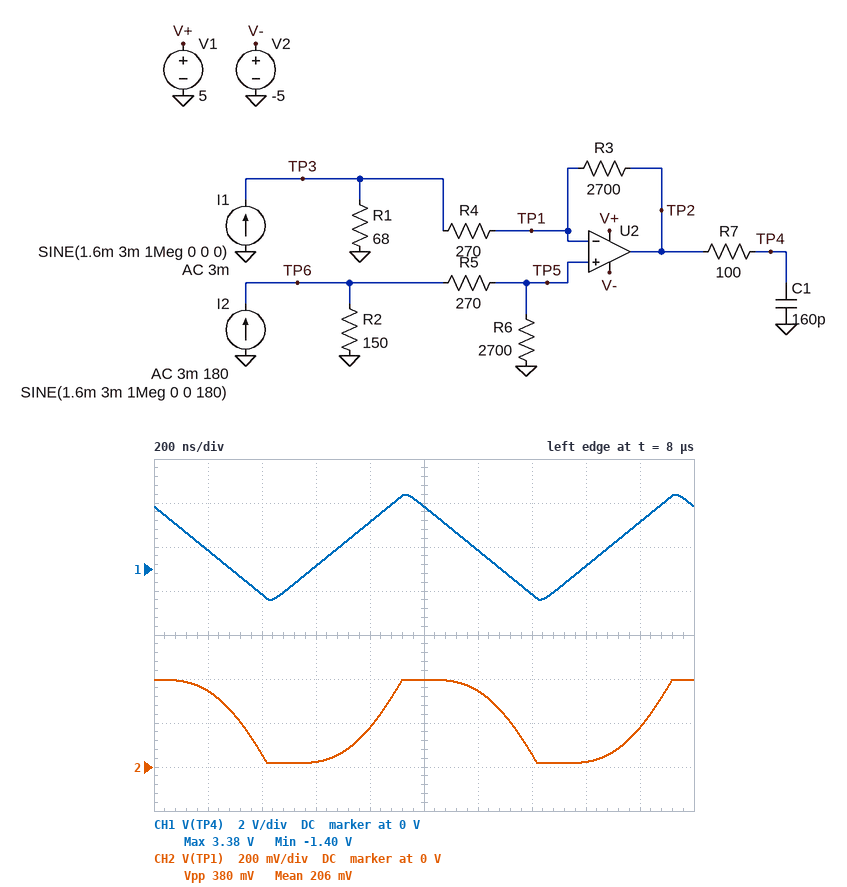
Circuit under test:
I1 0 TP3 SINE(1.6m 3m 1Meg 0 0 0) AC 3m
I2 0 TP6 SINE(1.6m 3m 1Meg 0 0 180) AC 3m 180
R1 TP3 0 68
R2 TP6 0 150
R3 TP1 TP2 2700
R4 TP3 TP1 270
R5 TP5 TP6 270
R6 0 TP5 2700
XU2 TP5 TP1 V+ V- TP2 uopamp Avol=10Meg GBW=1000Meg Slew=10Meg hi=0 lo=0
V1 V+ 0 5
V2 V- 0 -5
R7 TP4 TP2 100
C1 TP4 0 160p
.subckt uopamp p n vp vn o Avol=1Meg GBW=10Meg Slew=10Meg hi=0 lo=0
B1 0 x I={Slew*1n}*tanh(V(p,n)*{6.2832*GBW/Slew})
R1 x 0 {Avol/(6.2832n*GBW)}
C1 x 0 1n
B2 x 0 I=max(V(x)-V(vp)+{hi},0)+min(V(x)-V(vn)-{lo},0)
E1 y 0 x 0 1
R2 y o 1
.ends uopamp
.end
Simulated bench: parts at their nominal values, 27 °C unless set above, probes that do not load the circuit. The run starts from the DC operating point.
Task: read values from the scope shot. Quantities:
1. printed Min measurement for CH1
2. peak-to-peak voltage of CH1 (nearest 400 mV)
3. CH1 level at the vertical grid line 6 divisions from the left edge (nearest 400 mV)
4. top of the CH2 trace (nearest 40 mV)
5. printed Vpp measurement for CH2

-1.40 V
4.8 V
800 mV
400 mV
380 mV
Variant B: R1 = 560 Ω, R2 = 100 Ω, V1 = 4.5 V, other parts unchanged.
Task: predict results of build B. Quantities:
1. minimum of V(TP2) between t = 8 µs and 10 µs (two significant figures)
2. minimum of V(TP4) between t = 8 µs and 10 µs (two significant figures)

-4.8 V
-4.7 V
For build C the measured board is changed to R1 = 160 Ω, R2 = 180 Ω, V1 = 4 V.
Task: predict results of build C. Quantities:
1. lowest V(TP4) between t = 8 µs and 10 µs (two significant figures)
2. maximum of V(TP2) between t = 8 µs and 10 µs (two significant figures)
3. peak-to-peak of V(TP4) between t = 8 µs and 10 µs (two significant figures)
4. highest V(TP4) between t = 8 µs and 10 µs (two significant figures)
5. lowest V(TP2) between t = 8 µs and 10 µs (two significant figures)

-2.2 V
2.7 V
4.8 V
2.6 V
-2.3 V
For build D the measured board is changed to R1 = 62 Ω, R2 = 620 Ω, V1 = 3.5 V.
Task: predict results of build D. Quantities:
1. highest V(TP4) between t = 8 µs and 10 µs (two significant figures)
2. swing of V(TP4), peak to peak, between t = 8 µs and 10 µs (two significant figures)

3.5 V
3.9 V
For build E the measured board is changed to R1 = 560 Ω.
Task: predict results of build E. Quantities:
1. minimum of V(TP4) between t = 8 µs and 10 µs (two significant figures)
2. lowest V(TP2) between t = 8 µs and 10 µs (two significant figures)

-4.4 V
-4.5 V
